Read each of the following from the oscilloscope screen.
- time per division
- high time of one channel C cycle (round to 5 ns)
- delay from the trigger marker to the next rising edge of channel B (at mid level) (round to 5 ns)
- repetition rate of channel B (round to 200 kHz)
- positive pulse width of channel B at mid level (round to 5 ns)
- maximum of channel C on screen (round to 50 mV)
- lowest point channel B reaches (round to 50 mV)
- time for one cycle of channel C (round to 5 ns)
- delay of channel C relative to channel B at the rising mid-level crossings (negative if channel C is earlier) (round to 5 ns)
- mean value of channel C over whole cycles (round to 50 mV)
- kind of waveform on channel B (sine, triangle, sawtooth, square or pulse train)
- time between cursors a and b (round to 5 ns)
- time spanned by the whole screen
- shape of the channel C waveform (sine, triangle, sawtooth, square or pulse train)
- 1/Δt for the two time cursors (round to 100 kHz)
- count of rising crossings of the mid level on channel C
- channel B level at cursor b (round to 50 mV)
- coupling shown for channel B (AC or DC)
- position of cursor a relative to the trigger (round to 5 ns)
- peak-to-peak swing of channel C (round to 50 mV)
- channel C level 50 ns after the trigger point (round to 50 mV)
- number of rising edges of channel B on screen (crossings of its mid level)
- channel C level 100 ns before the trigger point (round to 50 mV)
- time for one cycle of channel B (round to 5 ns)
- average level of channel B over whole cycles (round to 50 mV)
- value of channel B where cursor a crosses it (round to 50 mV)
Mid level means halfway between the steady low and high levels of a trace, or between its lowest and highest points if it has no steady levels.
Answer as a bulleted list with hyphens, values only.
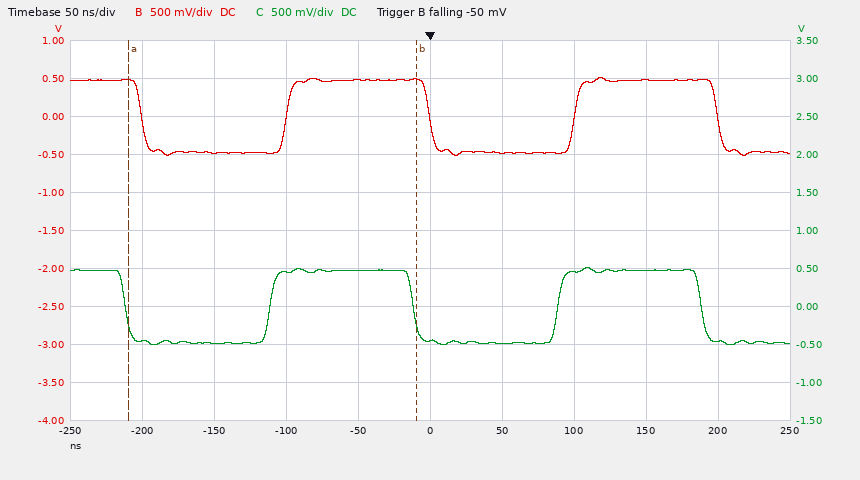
- 50 ns
- 100 ns
- 100 ns
- 5.0 MHz
- 100 ns
- 500 mV
- -500 mV
- 200 ns
- -10 ns
- 0 mV
- square
- 200 ns
- 500 ns
- square
- 5.0 MHz
- 2
- 500 mV
- DC
- -210 ns
- 1.00 V
- -500 mV
- 2
- 450 mV
- 200 ns
- 0 mV
- 500 mV
